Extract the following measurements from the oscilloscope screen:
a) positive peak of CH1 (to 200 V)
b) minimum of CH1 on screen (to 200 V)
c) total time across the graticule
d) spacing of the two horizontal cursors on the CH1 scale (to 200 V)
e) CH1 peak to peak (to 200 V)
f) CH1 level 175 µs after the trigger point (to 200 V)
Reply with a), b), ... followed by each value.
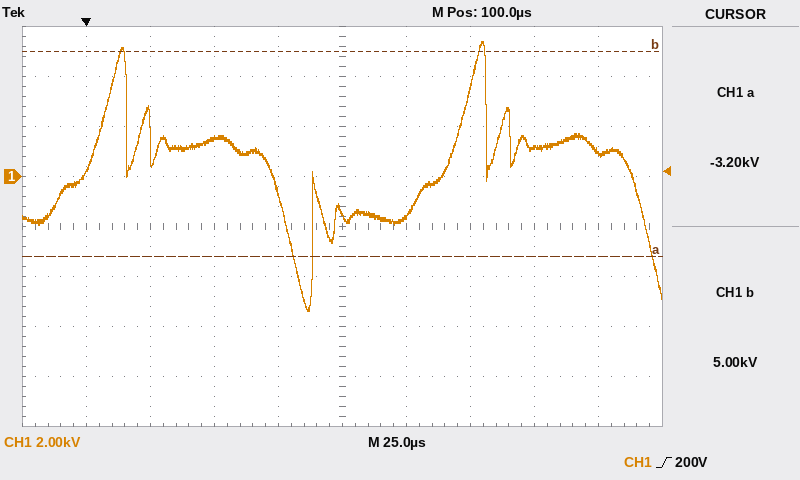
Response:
a) 5.4 kV
b) -5.4 kV
c) 250 µs
d) 8.2 kV
e) 10.8 kV
f) 1.2 kV
